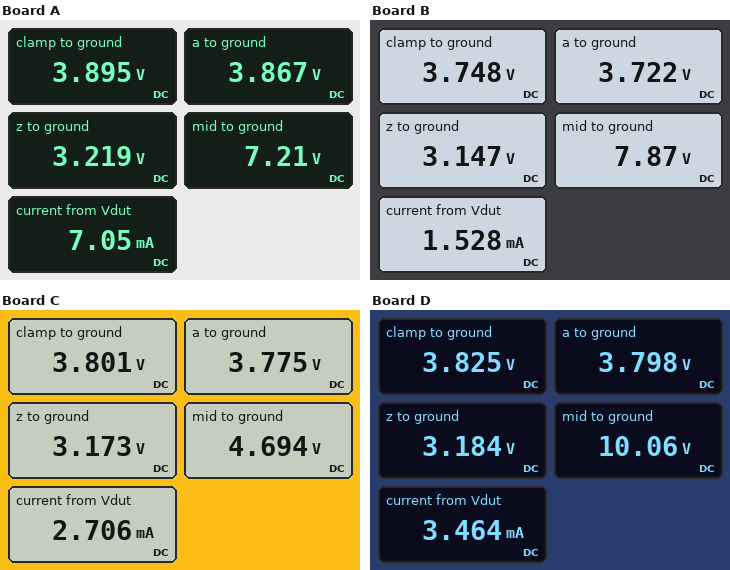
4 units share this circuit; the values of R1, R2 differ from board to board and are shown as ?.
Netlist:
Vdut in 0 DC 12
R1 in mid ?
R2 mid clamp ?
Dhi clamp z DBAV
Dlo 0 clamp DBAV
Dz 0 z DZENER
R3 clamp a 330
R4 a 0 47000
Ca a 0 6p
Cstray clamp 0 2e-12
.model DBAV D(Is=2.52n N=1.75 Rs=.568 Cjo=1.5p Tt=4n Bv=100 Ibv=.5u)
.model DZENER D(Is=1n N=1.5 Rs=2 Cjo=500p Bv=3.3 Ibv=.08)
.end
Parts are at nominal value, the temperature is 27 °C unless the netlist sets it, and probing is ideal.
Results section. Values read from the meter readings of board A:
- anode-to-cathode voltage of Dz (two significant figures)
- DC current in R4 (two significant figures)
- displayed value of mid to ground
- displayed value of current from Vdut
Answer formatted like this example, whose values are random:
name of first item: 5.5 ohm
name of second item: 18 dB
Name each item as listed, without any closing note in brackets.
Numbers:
anode-to-cathode voltage of Dz: -3.2 V
DC current in R4: 82 µA
displayed value of mid to ground: 7.21 V
displayed value of current from Vdut: 7.05 mA
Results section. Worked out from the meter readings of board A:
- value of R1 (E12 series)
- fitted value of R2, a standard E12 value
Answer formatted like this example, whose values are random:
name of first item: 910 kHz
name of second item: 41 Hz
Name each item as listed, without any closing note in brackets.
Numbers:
value of R1: 680 Ω
fitted value of R2, a standard E12 value: 470 Ω
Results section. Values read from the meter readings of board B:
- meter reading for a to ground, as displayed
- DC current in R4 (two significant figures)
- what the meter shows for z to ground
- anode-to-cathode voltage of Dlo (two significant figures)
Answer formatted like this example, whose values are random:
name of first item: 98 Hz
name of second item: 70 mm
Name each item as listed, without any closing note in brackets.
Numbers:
meter reading for a to ground, as displayed: 3.722 V
DC current in R4: 79 µA
what the meter shows for z to ground: 3.147 V
anode-to-cathode voltage of Dlo: -3.7 V
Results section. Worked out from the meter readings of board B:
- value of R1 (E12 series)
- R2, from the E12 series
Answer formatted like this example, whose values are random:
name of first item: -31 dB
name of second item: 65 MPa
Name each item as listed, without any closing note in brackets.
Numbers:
value of R1: 2.7 kΩ
R2, from the E12 series: 2.7 kΩ
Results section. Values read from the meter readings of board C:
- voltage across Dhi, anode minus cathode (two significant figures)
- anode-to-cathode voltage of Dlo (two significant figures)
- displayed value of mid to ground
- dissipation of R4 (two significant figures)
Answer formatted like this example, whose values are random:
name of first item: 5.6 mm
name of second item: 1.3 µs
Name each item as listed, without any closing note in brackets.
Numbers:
voltage across Dhi, anode minus cathode: 630 mV
anode-to-cathode voltage of Dlo: -3.8 V
displayed value of mid to ground: 4.694 V
dissipation of R4: 300 µW
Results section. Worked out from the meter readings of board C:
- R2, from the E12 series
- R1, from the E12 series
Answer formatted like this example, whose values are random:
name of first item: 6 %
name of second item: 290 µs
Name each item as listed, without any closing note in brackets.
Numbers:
R2, from the E12 series: 330 Ω
R1, from the E12 series: 2.7 kΩ
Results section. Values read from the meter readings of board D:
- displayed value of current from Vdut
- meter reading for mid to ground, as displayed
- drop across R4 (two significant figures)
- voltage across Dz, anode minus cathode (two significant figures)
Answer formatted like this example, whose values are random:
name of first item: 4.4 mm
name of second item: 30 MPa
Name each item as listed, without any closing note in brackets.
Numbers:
displayed value of current from Vdut: 3.464 mA
meter reading for mid to ground, as displayed: 10.06 V
drop across R4: 3.8 V
voltage across Dz, anode minus cathode: -3.2 V
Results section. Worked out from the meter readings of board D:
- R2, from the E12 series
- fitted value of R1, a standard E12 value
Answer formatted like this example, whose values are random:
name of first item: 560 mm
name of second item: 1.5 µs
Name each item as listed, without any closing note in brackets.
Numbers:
R2, from the E12 series: 1.8 kΩ
fitted value of R1, a standard E12 value: 560 Ω
